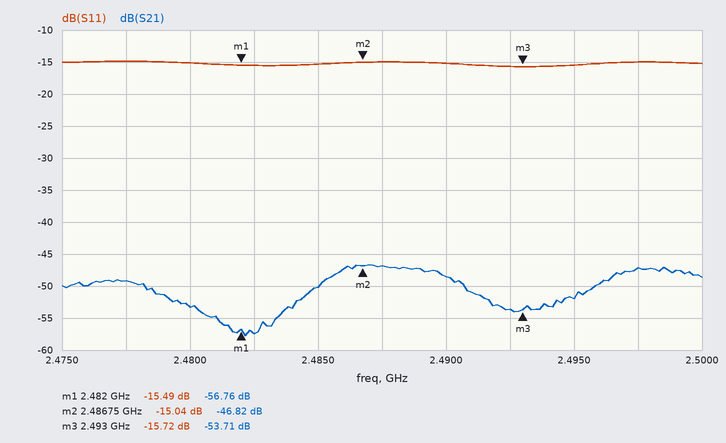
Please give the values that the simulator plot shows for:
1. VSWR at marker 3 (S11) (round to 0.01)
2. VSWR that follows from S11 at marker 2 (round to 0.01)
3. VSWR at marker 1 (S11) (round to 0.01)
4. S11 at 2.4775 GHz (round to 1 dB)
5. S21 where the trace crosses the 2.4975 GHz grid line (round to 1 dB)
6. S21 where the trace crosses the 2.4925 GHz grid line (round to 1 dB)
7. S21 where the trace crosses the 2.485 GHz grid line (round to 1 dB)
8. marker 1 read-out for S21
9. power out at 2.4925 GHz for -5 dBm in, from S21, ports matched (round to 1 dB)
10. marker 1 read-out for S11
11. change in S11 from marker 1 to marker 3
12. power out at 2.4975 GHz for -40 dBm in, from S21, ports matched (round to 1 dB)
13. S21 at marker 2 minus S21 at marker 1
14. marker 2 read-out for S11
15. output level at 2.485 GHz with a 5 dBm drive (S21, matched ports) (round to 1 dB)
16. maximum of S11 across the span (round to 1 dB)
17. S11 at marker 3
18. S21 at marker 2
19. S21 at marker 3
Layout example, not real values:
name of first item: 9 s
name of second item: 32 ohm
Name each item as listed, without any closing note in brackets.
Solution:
VSWR at marker 3 (S11): 1.39
VSWR that follows from S11 at marker 2: 1.43
VSWR at marker 1 (S11): 1.40
S11 at 2.4775 GHz: -15 dB
S21 where the trace crosses the 2.4975 GHz grid line: -47 dB
S21 where the trace crosses the 2.4925 GHz grid line: -54 dB
S21 where the trace crosses the 2.485 GHz grid line: -50 dB
marker 1 read-out for S21: -56.76 dB
power out at 2.4925 GHz for -5 dBm in, from S21, ports matched: -59 dBm
marker 1 read-out for S11: -15.49 dB
change in S11 from marker 1 to marker 3: -0.23 dB
power out at 2.4975 GHz for -40 dBm in, from S21, ports matched: -87 dBm
S21 at marker 2 minus S21 at marker 1: 9.94 dB
marker 2 read-out for S11: -15.04 dB
output level at 2.485 GHz with a 5 dBm drive (S21, matched ports): -45 dBm
maximum of S11 across the span: -15 dB
S11 at marker 3: -15.72 dB
S21 at marker 2: -46.82 dB
S21 at marker 3: -53.71 dB
